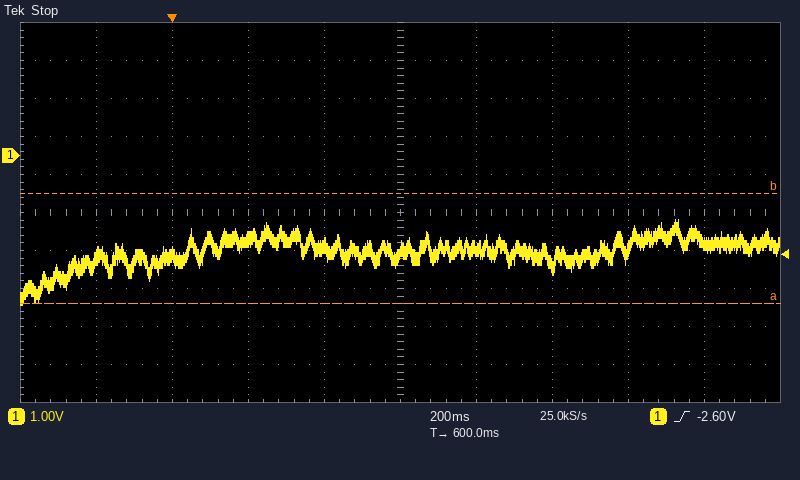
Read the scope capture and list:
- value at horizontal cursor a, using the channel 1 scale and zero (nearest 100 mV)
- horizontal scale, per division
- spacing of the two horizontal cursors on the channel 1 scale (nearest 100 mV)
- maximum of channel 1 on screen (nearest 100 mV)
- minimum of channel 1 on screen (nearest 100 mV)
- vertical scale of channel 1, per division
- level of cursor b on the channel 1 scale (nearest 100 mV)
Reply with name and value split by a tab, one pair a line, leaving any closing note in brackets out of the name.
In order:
value at horizontal cursor a, using the channel 1 scale and zero	-3.9 V
horizontal scale, per division	200 ms
spacing of the two horizontal cursors on the channel 1 scale	2.9 V
maximum of channel 1 on screen	-1.7 V
minimum of channel 1 on screen	-3.9 V
vertical scale of channel 1, per division	1 V
level of cursor b on the channel 1 scale	-1.0 V
